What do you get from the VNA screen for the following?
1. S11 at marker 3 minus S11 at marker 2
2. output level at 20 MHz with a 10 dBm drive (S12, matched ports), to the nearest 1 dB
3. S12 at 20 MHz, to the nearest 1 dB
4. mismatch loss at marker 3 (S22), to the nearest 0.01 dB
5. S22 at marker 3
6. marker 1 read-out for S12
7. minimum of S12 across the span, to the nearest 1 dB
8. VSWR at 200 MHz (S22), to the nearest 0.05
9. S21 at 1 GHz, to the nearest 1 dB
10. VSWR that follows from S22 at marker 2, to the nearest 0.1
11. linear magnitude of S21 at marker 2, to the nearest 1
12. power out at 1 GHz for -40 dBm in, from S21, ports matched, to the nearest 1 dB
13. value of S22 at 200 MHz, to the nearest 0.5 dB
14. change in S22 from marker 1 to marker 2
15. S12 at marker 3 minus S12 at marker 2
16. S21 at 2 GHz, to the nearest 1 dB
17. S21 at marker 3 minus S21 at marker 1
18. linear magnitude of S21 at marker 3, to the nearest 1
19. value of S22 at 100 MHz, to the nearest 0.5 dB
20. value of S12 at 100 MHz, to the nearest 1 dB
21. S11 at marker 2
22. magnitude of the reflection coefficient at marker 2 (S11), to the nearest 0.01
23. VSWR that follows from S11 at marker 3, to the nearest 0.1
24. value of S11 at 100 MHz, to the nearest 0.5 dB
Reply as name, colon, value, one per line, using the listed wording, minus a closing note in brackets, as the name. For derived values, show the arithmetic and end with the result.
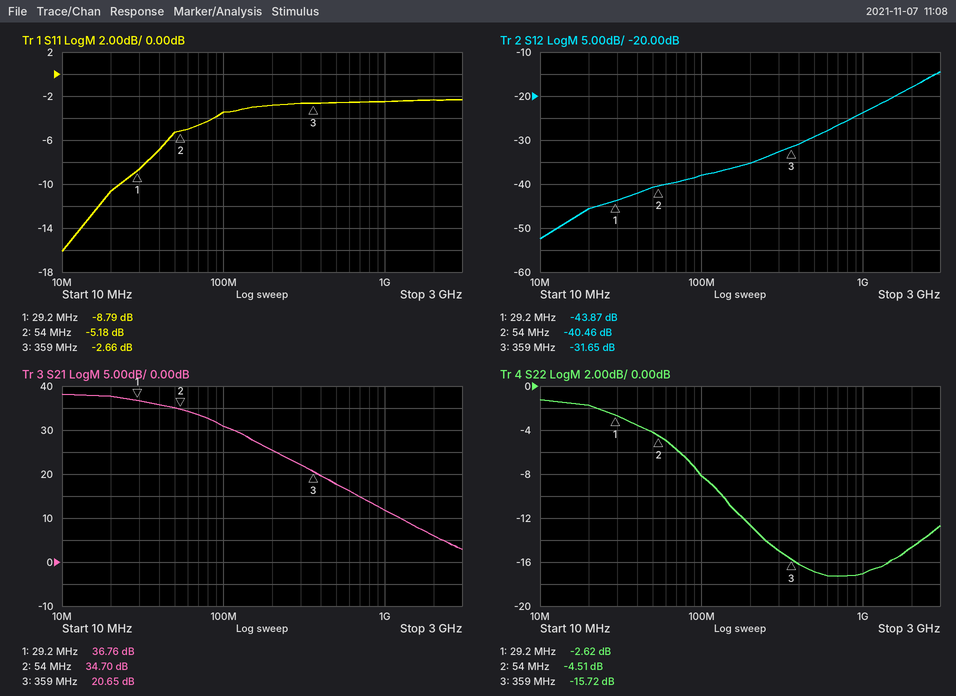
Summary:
S11 at marker 3 minus S11 at marker 2: -2.66 − (-5.18) = 2.52 dB
output level at 20 MHz with a 10 dBm drive (S12, matched ports), to the nearest 1 dB: 10 dBm + (-46 dB) = -36 dBm
S12 at 20 MHz, to the nearest 1 dB: -46 dB
mismatch loss at marker 3 (S22), to the nearest 0.01 dB: −10 log10(1 − 10^(-15.72/10)) ≈ 0.12 dB
S22 at marker 3: -15.72 dB
marker 1 read-out for S12: -43.87 dB
minimum of S12 across the span, to the nearest 1 dB: -52 dB
VSWR at 200 MHz (S22), to the nearest 0.05: |Γ| = 10^(-12.5/20) = 0.2371; VSWR = (1 + 0.2371)/(1 − 0.2371) ≈ 1.62, so 1.60 to the nearest 0.05
S21 at 1 GHz, to the nearest 1 dB: 12 dB
VSWR that follows from S22 at marker 2, to the nearest 0.1: (1 + 0.5950)/(1 − 0.5950) ≈ 3.9
linear magnitude of S21 at marker 2, to the nearest 1: 10^(34.7/20) ≈ 54
power out at 1 GHz for -40 dBm in, from S21, ports matched, to the nearest 1 dB: -40 dBm + (12 dB) = -28 dBm
value of S22 at 200 MHz, to the nearest 0.5 dB: -12.5 dB
change in S22 from marker 1 to marker 2: -4.51 − (-2.62) = -1.89 dB
S12 at marker 3 minus S12 at marker 2: -31.65 − (-40.46) = 8.81 dB
S21 at 2 GHz, to the nearest 1 dB: 6 dB
S21 at marker 3 minus S21 at marker 1: 20.65 − (36.76) = -16.11 dB
linear magnitude of S21 at marker 3, to the nearest 1: 10^(20.65/20) ≈ 11
value of S22 at 100 MHz, to the nearest 0.5 dB: -8.0 dB
value of S12 at 100 MHz, to the nearest 1 dB: -38 dB
S11 at marker 2: -5.18 dB
magnitude of the reflection coefficient at marker 2 (S11), to the nearest 0.01: 10^(-5.18/20) ≈ 0.55
VSWR that follows from S11 at marker 3, to the nearest 0.1: (1 + 0.7362)/(1 − 0.7362) ≈ 6.6
value of S11 at 100 MHz, to the nearest 0.5 dB: -3.5 dB
